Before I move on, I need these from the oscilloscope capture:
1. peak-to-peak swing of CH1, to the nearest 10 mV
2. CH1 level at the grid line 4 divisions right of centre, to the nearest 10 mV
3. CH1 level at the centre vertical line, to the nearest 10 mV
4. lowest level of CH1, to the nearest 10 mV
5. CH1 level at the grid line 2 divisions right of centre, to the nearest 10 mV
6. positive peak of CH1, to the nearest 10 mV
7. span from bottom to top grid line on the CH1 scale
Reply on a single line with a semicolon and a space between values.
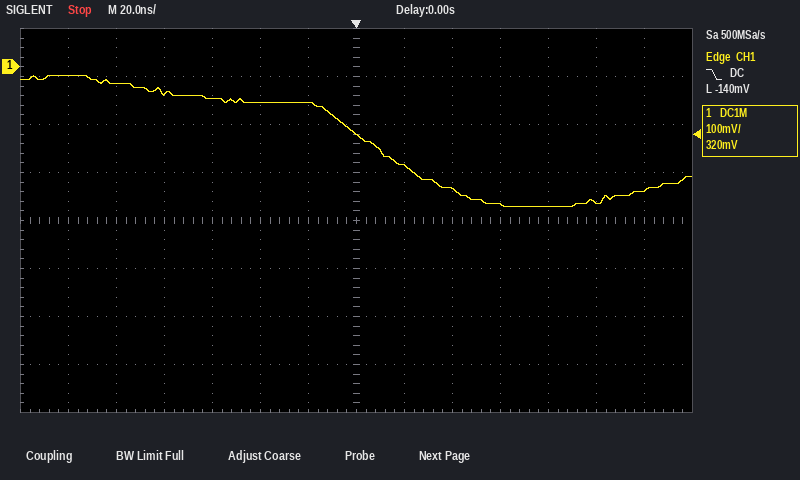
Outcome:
270 mV; -290 mV; -140 mV; -290 mV; -250 mV; -20 mV; 800 mV
